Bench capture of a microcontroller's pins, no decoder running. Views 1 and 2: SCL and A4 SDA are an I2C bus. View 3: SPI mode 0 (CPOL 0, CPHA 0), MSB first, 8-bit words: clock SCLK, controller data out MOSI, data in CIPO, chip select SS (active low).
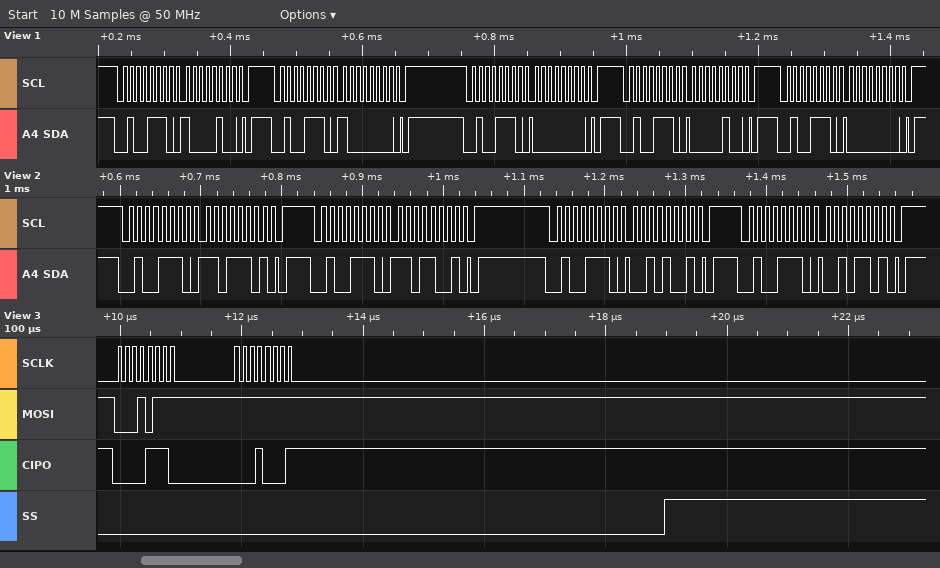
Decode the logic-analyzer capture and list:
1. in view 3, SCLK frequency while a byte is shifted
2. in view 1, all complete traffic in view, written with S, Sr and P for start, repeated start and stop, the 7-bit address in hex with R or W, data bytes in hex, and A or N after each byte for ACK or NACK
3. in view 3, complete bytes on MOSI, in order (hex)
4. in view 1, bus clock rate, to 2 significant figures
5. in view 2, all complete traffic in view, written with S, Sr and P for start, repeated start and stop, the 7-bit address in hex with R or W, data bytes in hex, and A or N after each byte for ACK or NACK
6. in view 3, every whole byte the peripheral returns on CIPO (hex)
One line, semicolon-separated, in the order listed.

8 MHz; S 27W A 84 A P S 27W A 80 A P S 27W A 00 A P S 27W A 04 A P S 27W A 00 A P; 0x17 0xFF; 100 kHz; S 27W A DD A P S 27W A D9 A P S 27W A 29 A P S 27W A 2D A P; 0x0E 0x11
